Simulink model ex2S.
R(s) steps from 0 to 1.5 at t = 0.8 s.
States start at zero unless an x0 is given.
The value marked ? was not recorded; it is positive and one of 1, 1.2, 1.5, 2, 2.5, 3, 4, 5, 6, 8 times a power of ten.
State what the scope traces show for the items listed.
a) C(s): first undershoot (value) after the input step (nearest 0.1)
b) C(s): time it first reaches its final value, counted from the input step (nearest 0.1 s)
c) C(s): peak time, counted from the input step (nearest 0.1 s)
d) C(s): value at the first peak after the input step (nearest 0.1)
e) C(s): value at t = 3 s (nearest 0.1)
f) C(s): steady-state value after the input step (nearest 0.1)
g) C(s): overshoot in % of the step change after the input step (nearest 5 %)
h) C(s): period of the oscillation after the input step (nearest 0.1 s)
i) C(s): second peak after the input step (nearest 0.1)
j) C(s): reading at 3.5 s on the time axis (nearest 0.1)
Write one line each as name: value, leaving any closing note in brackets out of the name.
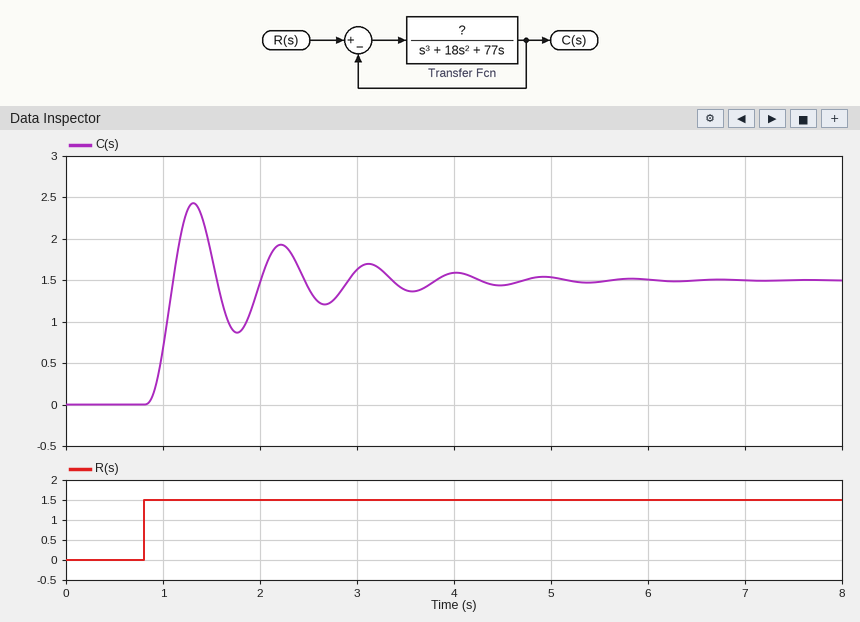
C(s): first undershoot (value) after the input step: 0.9
C(s): time it first reaches its final value, counted from the input step: 0.3 s
C(s): peak time, counted from the input step: 0.5 s
C(s): value at the first peak after the input step: 2.4
C(s): value at t = 3 s: 1.6
C(s): steady-state value after the input step: 1.5
C(s): overshoot in % of the step change after the input step: 60 %
C(s): period of the oscillation after the input step: 0.9 s
C(s): second peak after the input step: 1.9
C(s): reading at 3.5 s on the time axis: 1.4
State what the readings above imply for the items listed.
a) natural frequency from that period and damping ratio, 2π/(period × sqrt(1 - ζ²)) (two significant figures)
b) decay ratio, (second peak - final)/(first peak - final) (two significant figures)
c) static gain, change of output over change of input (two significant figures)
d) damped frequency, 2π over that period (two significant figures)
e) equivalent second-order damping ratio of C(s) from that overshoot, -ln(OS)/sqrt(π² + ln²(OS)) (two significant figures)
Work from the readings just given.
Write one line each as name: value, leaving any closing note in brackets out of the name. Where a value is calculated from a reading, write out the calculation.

natural frequency from that period and damping ratio, 2π/(period × sqrt(1 - ζ²)): 2π / (0.9 × sqrt(1 - 0.16²)) = 7.1 rad/s
decay ratio, (second peak - final)/(first peak - final): (1.9 - 1.5) / (2.4 - 1.5) = 0.44
static gain, change of output over change of input: (1.5 - 0) / (1.5 - 0) = 1.0
damped frequency, 2π over that period: 2π / 0.9 = 7.0 rad/s
equivalent second-order damping ratio of C(s) from that overshoot, -ln(OS)/sqrt(π² + ln²(OS)): ln(0.6) = -0.511; 0.511 / sqrt(9.870 + 0.261) = 0.16
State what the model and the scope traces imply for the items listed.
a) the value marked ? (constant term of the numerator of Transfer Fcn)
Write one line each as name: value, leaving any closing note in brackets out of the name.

the value marked ?: 800
